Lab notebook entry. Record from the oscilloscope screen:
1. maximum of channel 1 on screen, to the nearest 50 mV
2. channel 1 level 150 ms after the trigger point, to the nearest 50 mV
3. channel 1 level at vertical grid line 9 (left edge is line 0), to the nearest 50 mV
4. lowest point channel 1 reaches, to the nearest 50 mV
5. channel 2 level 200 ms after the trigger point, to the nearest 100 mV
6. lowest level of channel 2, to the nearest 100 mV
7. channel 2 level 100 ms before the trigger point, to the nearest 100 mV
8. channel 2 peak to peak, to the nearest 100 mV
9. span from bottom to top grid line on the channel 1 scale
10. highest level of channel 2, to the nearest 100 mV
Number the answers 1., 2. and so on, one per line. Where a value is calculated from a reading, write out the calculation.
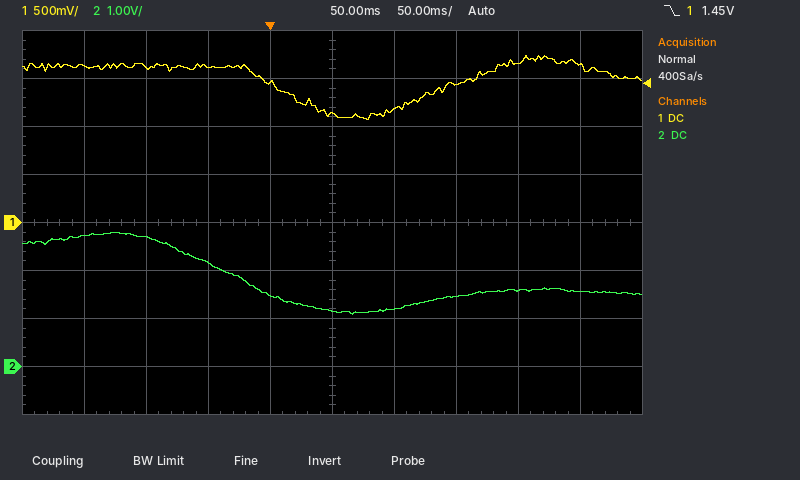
1. 1.75 V
2. 1.45 V
3. 1.65 V
4. 1.05 V
5. 1.6 V
6. 1.1 V
7. 2.7 V
8. 2.8 V − (1.1 V) = 1.7 V
9. 4 V
10. 2.8 V
